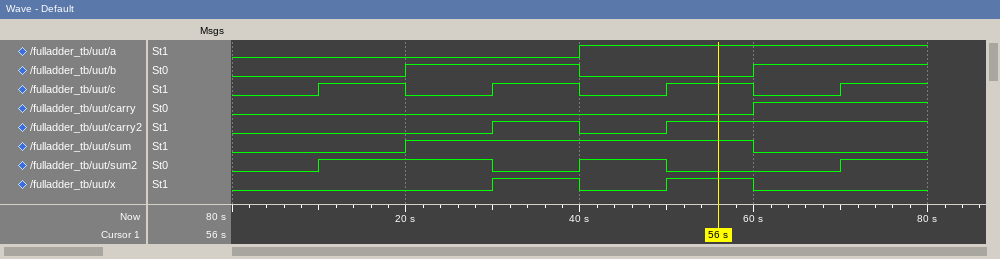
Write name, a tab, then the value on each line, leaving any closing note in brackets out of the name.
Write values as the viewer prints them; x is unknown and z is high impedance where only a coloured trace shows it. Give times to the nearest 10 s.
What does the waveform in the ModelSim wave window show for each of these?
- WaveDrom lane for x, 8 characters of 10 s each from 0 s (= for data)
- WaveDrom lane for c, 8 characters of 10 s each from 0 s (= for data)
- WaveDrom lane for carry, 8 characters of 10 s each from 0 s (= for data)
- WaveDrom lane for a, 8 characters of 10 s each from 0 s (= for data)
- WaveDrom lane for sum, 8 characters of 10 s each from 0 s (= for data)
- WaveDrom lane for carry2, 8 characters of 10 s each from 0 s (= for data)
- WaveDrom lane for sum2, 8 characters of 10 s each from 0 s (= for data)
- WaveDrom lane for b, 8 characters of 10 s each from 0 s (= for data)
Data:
WaveDrom lane for x, 8 characters of 10 s each from 0 s	{name: 'x', wave: '0..1010.'}
WaveDrom lane for c, 8 characters of 10 s each from 0 s	{name: 'c', wave: '01010101'}
WaveDrom lane for carry, 8 characters of 10 s each from 0 s	{name: 'carry', wave: '0.....1.'}
WaveDrom lane for a, 8 characters of 10 s each from 0 s	{name: 'a', wave: '0...1...'}
WaveDrom lane for sum, 8 characters of 10 s each from 0 s	{name: 'sum', wave: '0.1...0.'}
WaveDrom lane for carry2, 8 characters of 10 s each from 0 s	{name: 'carry2', wave: '0..101..'}
WaveDrom lane for sum2, 8 characters of 10 s each from 0 s	{name: 'sum2', wave: '01.010.1'}
WaveDrom lane for b, 8 characters of 10 s each from 0 s	{name: 'b', wave: '0.1.0.1.'}
